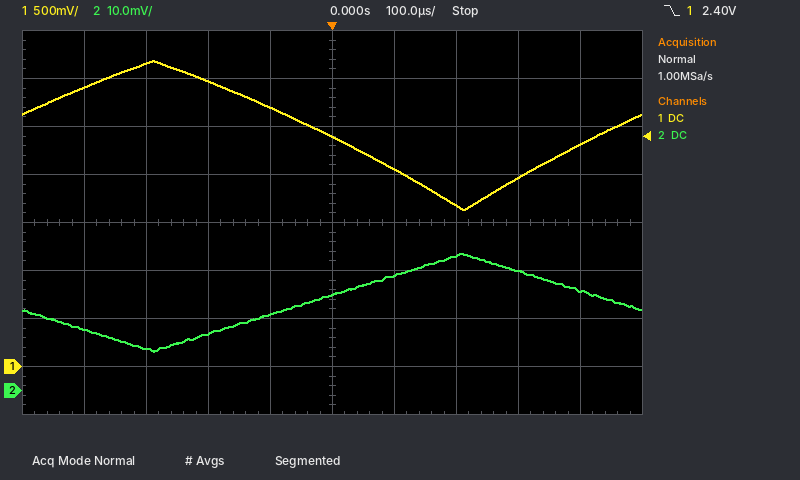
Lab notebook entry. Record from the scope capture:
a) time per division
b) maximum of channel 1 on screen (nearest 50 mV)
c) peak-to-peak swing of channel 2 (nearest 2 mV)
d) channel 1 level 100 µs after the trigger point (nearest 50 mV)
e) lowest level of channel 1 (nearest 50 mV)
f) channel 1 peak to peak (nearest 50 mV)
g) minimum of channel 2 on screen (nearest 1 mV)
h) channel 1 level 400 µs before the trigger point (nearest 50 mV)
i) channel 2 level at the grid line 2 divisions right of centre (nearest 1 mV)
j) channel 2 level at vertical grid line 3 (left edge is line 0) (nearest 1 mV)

100 µs
3.20 V
20 mV
2.05 V
1.65 V
1.55 V
8 mV
2.90 V
28 mV
12 mV
